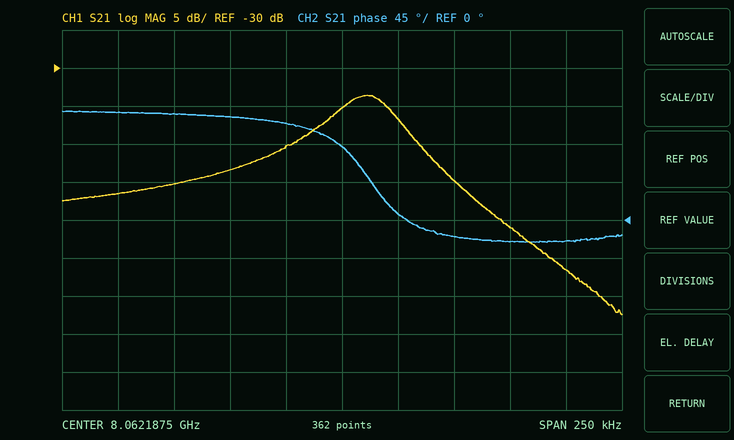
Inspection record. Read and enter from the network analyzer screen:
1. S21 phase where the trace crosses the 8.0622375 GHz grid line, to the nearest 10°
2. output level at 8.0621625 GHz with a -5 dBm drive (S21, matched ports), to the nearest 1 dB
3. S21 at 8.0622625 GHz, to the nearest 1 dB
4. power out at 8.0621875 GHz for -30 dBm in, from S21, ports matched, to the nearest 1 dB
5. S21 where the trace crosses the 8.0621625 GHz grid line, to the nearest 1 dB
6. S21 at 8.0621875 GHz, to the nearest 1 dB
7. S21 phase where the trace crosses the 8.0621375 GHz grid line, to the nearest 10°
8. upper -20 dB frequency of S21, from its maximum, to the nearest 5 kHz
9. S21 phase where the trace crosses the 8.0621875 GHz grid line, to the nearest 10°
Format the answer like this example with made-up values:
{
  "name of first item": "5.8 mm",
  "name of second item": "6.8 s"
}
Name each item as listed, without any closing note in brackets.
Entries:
{
  "S21 phase where the trace crosses the 8.0622375 GHz grid line, to the nearest 10°": "-20°",
  "output level at 8.0621625 GHz with a -5 dBm drive (S21, matched ports), to the nearest 1 dB": "-45 dBm",
  "S21 at 8.0622625 GHz, to the nearest 1 dB": "-51 dB",
  "power out at 8.0621875 GHz for -30 dBm in, from S21, ports matched, to the nearest 1 dB": "-65 dBm",
  "S21 where the trace crosses the 8.0621625 GHz grid line, to the nearest 1 dB": "-40 dB",
  "S21 at 8.0621875 GHz, to the nearest 1 dB": "-35 dB",
  "S21 phase where the trace crosses the 8.0621375 GHz grid line, to the nearest 10°": "120°",
  "upper -20 dB frequency of S21, from its maximum, to the nearest 5 kHz": "8.062275 GHz",
  "S21 phase where the trace crosses the 8.0621875 GHz grid line, to the nearest 10°": "90°"
}
